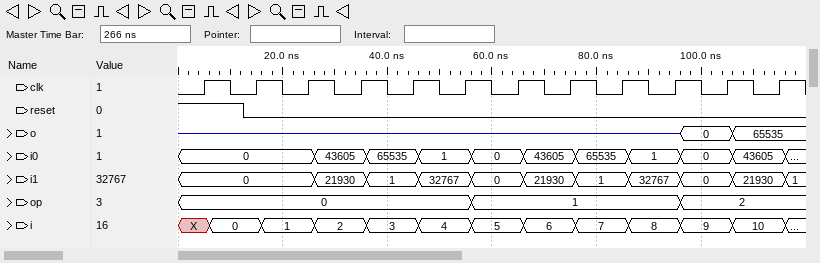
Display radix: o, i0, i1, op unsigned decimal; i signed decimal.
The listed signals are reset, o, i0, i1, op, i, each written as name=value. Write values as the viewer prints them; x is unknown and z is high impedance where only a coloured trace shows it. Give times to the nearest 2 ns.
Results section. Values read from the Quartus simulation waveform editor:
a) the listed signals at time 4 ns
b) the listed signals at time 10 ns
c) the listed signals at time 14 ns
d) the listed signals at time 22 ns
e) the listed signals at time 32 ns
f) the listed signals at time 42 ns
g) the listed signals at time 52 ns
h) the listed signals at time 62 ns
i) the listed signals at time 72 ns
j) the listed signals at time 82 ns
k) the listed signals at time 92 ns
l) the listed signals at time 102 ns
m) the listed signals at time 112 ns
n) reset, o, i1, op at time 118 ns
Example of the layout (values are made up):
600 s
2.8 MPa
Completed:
reset=1, o=z, i0=0, i1=0, op=0, i=X
reset=1, o=z, i0=0, i1=0, op=0, i=0
reset=0, o=z, i0=0, i1=0, op=0, i=0
reset=0, o=z, i0=0, i1=0, op=0, i=1
reset=0, o=z, i0=43605, i1=21930, op=0, i=2
reset=0, o=z, i0=65535, i1=1, op=0, i=3
reset=0, o=z, i0=1, i1=32767, op=0, i=4
reset=0, o=z, i0=0, i1=0, op=1, i=5
reset=0, o=z, i0=43605, i1=21930, op=1, i=6
reset=0, o=z, i0=65535, i1=1, op=1, i=7
reset=0, o=z, i0=1, i1=32767, op=1, i=8
reset=0, o=0, i0=0, i1=0, op=2, i=9
reset=0, o=65535, i0=43605, i1=21930, op=2, i=10
reset=0, o=65535, i1=1, op=2
